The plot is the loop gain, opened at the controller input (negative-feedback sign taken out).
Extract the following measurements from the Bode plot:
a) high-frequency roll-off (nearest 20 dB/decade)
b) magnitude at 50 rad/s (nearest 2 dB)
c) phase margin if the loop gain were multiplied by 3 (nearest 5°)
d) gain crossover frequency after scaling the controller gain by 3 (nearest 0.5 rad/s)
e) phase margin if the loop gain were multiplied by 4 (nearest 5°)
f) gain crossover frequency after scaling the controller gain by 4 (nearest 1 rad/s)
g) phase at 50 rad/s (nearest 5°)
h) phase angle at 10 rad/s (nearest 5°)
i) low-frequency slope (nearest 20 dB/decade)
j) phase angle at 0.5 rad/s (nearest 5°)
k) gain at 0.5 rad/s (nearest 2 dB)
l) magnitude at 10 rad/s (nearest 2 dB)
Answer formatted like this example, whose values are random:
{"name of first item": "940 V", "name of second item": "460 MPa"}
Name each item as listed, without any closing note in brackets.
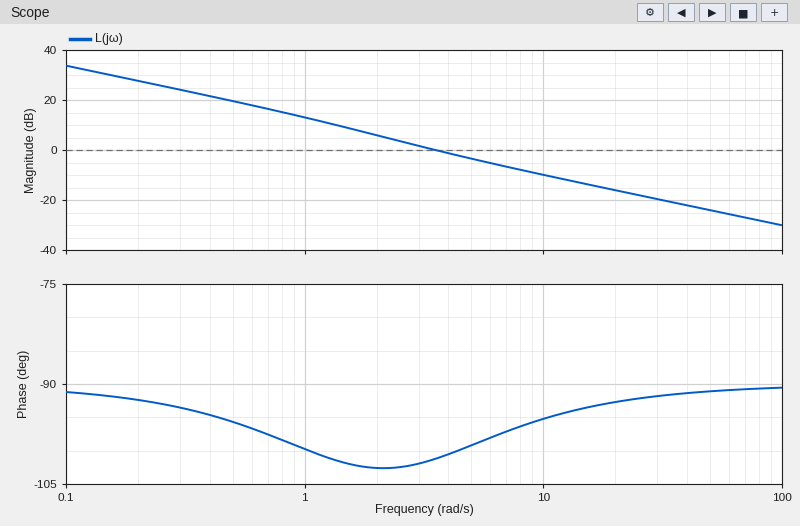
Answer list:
{"high-frequency roll-off": "-20 dB/decade", "magnitude at 50 rad/s": "-24 dB", "phase margin if the loop gain were multiplied by 3": "85°", "gain crossover frequency after scaling the controller gain by 3": "9.5 rad/s", "phase margin if the loop gain were multiplied by 4": "85°", "gain crossover frequency after scaling the controller gain by 4": "13 rad/s", "phase at 50 rad/s": "-90°", "phase angle at 10 rad/s": "-95°", "low-frequency slope": "-20 dB/decade", "phase angle at 0.5 rad/s": "-95°", "gain at 0.5 rad/s": "20 dB", "magnitude at 10 rad/s": "-10 dB"}
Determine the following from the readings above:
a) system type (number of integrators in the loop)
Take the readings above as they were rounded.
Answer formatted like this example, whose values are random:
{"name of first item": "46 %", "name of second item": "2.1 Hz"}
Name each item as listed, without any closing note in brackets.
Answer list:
{"system type": "1"}
